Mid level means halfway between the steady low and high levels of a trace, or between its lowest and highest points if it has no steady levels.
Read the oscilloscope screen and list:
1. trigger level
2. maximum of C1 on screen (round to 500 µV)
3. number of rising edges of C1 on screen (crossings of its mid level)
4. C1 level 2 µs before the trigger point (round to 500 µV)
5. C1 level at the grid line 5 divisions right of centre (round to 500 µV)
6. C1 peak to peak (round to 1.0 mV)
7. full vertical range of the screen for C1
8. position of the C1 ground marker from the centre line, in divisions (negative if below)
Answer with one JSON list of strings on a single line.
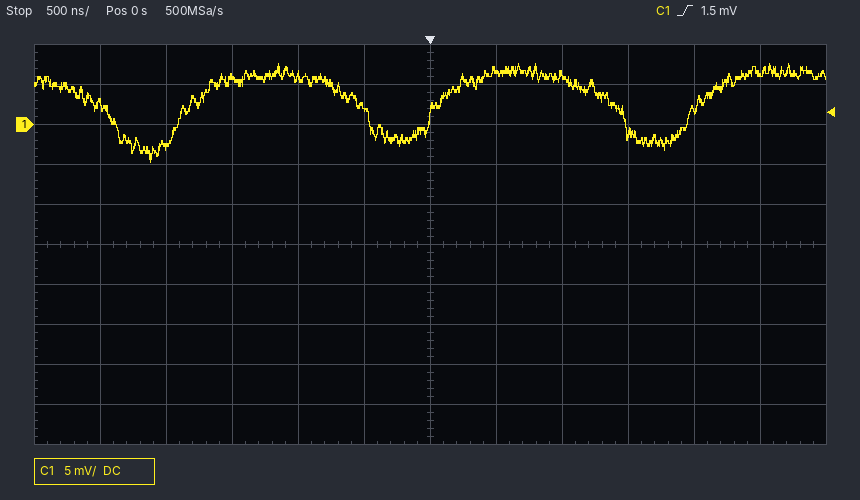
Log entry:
["1.5 mV", "7.5 mV", "3", "-3.0 mV", "6.5 mV", "12.0 mV", "50 mV", "+3.0 div"]
